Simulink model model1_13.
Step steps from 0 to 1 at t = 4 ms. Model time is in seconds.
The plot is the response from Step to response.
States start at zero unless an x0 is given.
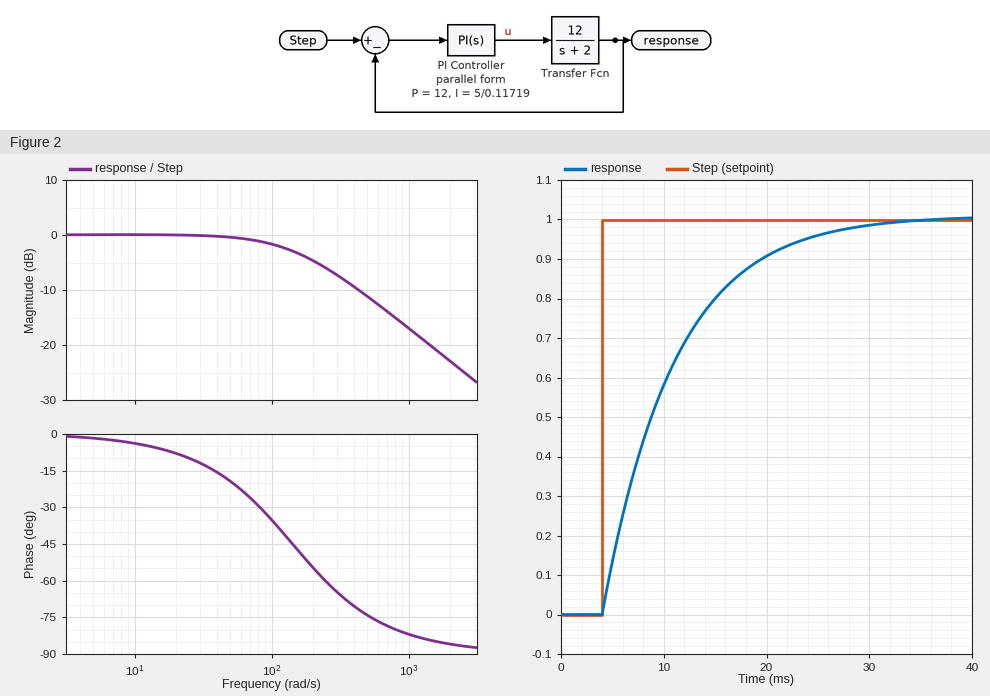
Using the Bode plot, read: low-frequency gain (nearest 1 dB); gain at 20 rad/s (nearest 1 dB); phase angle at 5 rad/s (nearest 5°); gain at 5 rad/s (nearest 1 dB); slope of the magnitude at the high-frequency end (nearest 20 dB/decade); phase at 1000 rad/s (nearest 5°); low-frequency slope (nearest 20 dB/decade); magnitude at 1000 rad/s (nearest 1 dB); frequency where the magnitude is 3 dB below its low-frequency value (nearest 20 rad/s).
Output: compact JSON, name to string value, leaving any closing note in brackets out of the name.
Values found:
{"low-frequency gain": "0 dB", "gain at 20 rad/s": "0 dB", "phase angle at 5 rad/s": "0°", "gain at 5 rad/s": "0 dB", "slope of the magnitude at the high-frequency end": "-20 dB/decade", "phase at 1000 rad/s": "-80°", "low-frequency slope": "0 dB/decade", "magnitude at 1000 rad/s": "-17 dB", "frequency where the magnitude is 3 dB below its low-frequency value": "140 rad/s"}
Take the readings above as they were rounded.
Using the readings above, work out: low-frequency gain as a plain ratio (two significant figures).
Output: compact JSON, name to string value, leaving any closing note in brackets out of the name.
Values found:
{"low-frequency gain as a plain ratio": "1.0"}
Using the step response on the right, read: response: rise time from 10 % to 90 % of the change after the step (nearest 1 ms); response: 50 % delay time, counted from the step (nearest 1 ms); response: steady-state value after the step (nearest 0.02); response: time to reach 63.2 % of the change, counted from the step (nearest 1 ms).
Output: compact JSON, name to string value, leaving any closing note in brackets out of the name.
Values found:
{"response: rise time from 10 % to 90 % of the change after the step": "15 ms", "response: 50 % delay time, counted from the step": "5 ms", "response: steady-state value after the step": "1.00", "response: time to reach 63.2 % of the change, counted from the step": "7 ms"}
